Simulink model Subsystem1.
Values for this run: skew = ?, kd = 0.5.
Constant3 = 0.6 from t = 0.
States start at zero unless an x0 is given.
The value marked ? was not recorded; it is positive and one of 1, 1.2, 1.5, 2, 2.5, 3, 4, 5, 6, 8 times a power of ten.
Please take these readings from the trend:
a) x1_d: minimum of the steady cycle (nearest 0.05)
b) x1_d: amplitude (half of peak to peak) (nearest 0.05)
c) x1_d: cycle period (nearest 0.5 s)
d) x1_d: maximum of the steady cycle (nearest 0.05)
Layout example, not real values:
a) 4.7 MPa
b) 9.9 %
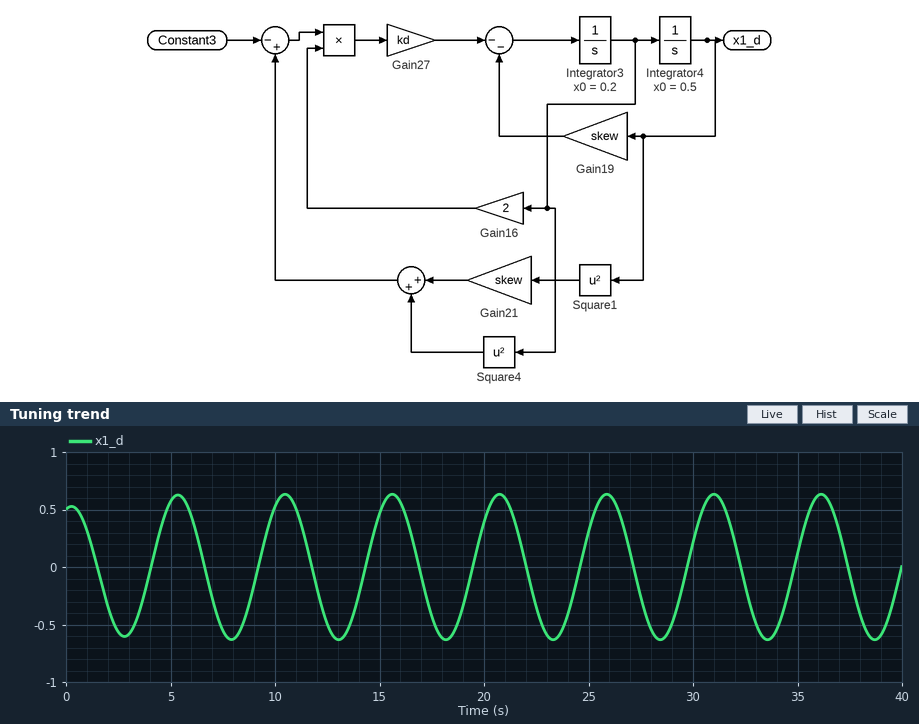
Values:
a) -0.65
b) 0.65
c) 5.0 s
d) 0.65
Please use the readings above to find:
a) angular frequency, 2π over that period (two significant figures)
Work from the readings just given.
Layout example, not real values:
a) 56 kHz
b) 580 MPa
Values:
a) 1.3 rad/s
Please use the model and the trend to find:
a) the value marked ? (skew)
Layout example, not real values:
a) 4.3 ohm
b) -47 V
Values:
a) 1.5
